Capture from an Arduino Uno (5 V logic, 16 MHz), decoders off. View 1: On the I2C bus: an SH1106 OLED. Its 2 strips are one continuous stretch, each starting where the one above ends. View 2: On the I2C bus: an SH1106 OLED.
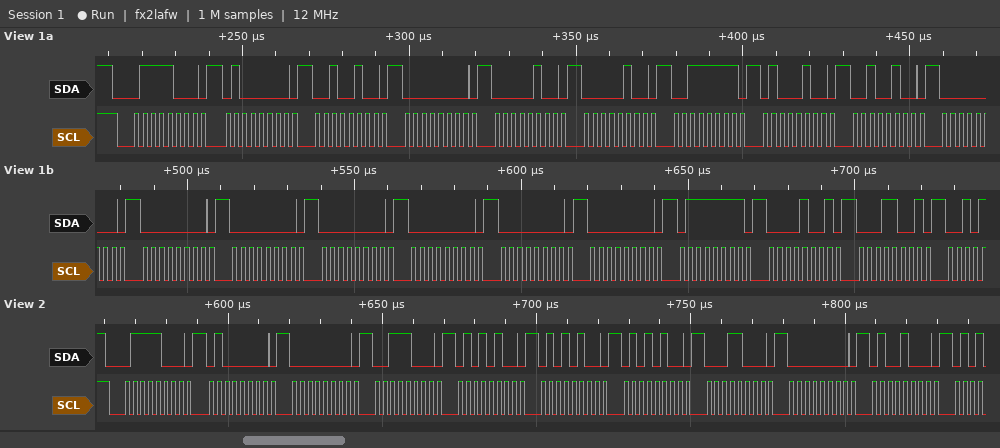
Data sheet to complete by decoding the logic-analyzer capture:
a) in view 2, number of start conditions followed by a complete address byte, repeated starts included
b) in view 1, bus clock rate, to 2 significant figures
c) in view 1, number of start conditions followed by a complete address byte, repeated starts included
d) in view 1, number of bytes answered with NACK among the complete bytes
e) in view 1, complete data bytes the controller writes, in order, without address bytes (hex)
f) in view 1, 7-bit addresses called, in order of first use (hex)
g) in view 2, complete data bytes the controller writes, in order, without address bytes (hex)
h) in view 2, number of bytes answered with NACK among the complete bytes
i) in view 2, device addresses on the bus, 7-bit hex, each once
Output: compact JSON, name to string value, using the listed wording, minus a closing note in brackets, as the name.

{"in view 2, number of start conditions followed by a complete address byte, repeated starts included": "1", "in view 1, bus clock rate, to 2 significant figures": "400 kHz", "in view 1, number of start conditions followed by a complete address byte, repeated starts included": "1", "in view 1, number of bytes answered with NACK among the complete bytes": "0", "in view 1, complete data bytes the controller writes, in order, without address bytes": "40 24 00 04 04 3F 44 24 00 00 00 00 00 00 00 7F 09 19", "in view 1, 7-bit addresses called, in order of first use": "0x3C", "in view 2, complete data bytes the controller writes, in order, without address bytes": "40 00 38 54 54 54 18 00 48", "in view 2, number of bytes answered with NACK among the complete bytes": "0", "in view 2, device addresses on the bus, 7-bit hex, each once": "0x3C"}
